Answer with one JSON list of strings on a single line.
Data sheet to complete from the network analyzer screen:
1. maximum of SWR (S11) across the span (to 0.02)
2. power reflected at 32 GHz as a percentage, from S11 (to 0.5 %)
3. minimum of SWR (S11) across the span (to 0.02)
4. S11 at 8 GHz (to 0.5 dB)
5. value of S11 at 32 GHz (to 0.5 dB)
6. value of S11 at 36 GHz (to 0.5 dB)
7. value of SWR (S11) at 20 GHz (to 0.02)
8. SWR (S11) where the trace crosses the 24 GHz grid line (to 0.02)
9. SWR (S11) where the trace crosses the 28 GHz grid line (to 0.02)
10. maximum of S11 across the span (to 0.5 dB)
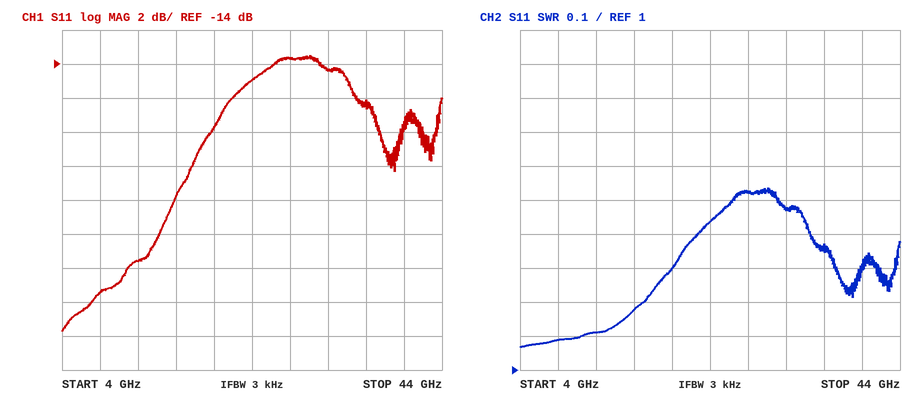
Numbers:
["1.54", "3.5 %", "1.06", "-27.5 dB", "-14.5 dB", "-16.5 dB", "1.30", "1.44", "1.52", "-13.5 dB"]
